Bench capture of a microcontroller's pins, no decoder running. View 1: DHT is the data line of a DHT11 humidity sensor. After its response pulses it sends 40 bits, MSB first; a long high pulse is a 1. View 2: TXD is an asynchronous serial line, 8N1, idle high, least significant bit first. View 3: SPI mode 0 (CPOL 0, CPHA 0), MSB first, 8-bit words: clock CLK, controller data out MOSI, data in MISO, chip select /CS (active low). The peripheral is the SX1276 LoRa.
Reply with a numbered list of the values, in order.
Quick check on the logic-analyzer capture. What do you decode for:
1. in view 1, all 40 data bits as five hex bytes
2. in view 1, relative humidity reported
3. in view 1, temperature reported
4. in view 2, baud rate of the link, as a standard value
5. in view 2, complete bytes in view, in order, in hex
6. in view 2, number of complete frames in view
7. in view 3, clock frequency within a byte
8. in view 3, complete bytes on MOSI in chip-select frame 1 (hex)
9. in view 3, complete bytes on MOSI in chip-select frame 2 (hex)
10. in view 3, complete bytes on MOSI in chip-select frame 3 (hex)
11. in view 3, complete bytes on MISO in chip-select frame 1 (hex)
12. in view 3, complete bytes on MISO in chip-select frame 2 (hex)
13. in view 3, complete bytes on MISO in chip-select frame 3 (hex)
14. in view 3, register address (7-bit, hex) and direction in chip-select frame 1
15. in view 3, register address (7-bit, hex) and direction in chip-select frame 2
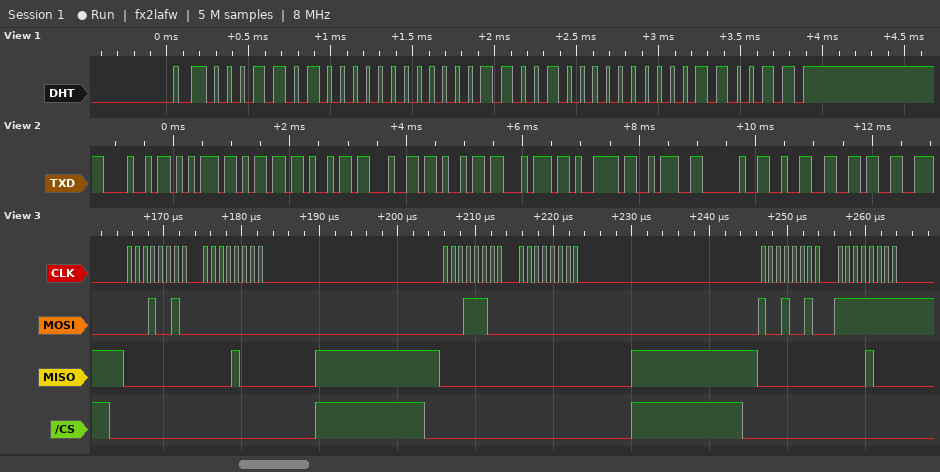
1. 1A 00 19 00 33
2. 26 %
3. 25.0 °C
4. 9600 baud
5. 48 75 6D 69 64 69 74 79 3A 20 32 36
6. 12
7. 1 MHz
8. 12 00
9. 1C 00
10. 92 FF
11. 00 08
12. 00 00
13. 00 08
14. 0x12 read
15. 0x1C read
